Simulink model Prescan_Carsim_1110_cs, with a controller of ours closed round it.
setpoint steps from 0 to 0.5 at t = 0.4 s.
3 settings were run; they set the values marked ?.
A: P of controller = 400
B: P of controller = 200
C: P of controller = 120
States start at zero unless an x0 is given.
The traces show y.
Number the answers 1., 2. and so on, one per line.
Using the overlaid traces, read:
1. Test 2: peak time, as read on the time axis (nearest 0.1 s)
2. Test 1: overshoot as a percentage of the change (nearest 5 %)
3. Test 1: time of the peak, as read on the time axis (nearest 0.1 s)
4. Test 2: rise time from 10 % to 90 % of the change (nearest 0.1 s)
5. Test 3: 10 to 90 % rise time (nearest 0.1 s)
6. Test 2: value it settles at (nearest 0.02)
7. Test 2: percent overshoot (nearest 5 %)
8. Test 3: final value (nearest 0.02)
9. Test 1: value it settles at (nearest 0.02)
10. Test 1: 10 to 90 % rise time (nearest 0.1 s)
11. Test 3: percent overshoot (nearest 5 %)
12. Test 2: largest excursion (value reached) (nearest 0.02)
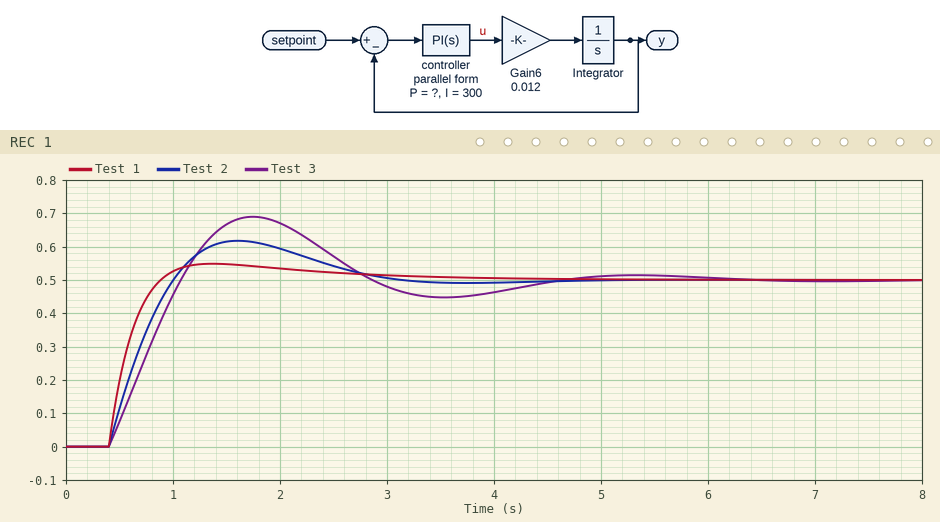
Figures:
1. 1.6 s
2. 10 %
3. 1.4 s
4. 0.5 s
5. 0.5 s
6. 0.50
7. 25 %
8. 0.50
9. 0.50
10. 0.3 s
11. 40 %
12. 0.62
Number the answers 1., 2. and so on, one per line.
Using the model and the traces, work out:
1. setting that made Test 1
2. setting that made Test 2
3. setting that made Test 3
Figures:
1. A
2. B
3. C
